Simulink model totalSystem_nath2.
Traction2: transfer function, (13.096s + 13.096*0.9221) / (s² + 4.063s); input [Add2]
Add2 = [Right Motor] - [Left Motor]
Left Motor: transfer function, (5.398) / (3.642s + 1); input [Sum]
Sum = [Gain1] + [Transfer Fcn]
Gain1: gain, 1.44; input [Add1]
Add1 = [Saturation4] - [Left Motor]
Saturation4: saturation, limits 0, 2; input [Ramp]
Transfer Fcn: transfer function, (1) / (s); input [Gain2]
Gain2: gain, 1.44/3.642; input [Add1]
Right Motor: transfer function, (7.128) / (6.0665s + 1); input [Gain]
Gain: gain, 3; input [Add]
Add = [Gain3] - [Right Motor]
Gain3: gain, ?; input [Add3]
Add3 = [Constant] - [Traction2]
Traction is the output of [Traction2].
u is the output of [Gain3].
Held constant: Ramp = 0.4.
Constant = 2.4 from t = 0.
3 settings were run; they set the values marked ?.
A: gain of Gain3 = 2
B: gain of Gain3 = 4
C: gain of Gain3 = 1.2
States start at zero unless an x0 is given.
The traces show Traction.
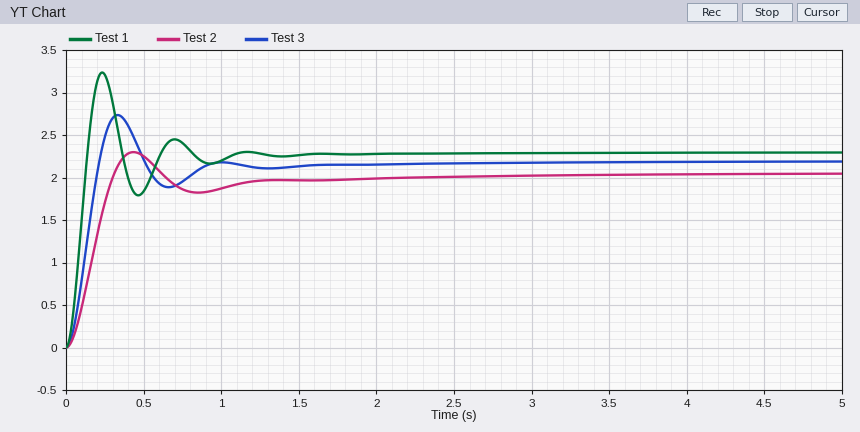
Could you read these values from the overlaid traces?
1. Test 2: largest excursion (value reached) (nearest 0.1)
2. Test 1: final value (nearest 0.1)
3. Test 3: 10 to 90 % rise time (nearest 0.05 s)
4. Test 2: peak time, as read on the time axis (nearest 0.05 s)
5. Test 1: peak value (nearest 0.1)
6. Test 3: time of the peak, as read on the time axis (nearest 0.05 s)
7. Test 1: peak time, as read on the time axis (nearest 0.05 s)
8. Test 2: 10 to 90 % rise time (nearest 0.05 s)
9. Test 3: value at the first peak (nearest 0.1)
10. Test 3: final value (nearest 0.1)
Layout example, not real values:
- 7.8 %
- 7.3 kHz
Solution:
- 2.3
- 2.3
- 0.15 s
- 0.45 s
- 3.2
- 0.35 s
- 0.25 s
- 0.20 s
- 2.7
- 2.2
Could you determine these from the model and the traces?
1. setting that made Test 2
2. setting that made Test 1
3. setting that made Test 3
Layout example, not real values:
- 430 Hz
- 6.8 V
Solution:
- C
- B
- A
